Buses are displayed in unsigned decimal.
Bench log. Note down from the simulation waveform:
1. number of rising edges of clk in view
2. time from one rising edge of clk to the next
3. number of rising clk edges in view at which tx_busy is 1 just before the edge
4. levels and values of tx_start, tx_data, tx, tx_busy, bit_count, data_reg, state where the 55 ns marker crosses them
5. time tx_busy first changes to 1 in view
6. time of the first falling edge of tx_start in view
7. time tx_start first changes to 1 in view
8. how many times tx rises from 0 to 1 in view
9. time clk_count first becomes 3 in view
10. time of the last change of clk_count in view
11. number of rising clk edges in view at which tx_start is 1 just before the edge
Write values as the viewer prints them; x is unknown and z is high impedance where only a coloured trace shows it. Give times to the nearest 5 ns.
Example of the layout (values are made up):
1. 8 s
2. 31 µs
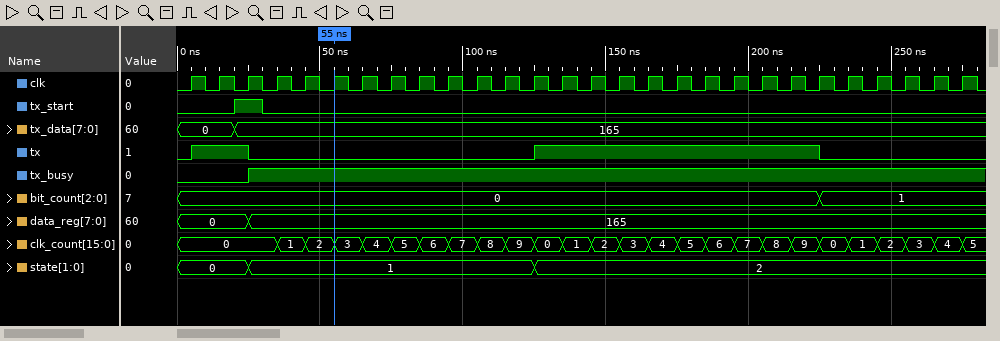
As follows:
1. 28
2. 10 ns
3. 25
4. tx_start=0, tx_data=165, tx=0, tx_busy=1, bit_count=0, data_reg=165, state=1
5. 25 ns
6. 30 ns
7. 20 ns
8. 2
9. 55 ns
10. 275 ns
11. 1
